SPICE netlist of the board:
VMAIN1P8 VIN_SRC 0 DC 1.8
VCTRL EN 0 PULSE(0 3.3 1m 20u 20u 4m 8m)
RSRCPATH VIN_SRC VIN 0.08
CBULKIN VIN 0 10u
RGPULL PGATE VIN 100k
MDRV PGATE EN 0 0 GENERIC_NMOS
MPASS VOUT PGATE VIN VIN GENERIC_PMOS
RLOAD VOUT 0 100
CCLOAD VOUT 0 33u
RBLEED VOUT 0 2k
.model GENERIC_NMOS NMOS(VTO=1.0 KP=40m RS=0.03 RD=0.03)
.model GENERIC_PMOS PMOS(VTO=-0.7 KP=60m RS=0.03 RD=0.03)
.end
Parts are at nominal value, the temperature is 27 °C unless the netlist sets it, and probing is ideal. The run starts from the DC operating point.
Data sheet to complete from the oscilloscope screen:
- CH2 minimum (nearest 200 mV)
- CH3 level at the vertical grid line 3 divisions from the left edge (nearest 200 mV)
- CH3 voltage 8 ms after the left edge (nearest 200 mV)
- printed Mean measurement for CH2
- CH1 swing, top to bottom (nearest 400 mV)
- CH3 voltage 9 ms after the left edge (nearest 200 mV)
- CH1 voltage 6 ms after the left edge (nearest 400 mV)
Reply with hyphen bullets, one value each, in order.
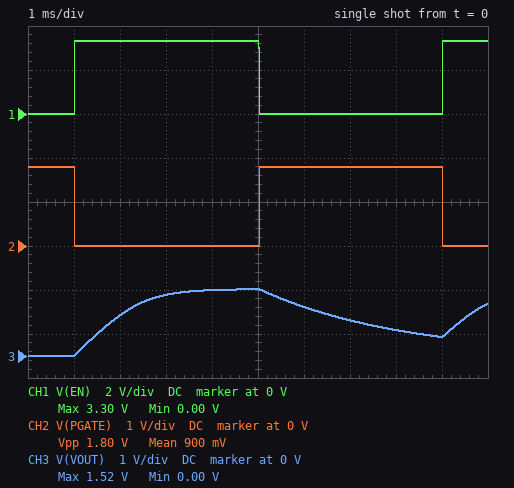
- 0 V
- 1.4 V
- 600 mV
- 900 mV
- 3.2 V
- 400 mV
- 0 V
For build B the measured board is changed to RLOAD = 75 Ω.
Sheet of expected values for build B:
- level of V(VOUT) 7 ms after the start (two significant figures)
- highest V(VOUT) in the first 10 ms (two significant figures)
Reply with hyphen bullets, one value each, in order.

- 630 mV
- 1.4 V
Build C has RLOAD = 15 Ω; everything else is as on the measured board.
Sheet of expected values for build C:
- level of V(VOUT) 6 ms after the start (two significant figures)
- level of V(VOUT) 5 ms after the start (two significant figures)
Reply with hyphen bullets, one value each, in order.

- 75 mV
- 540 mV
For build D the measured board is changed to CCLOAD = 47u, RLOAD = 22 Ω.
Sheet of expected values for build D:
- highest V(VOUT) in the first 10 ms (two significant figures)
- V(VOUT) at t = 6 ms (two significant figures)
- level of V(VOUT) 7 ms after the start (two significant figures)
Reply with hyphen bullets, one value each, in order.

- 770 mV
- 300 mV
- 110 mV
